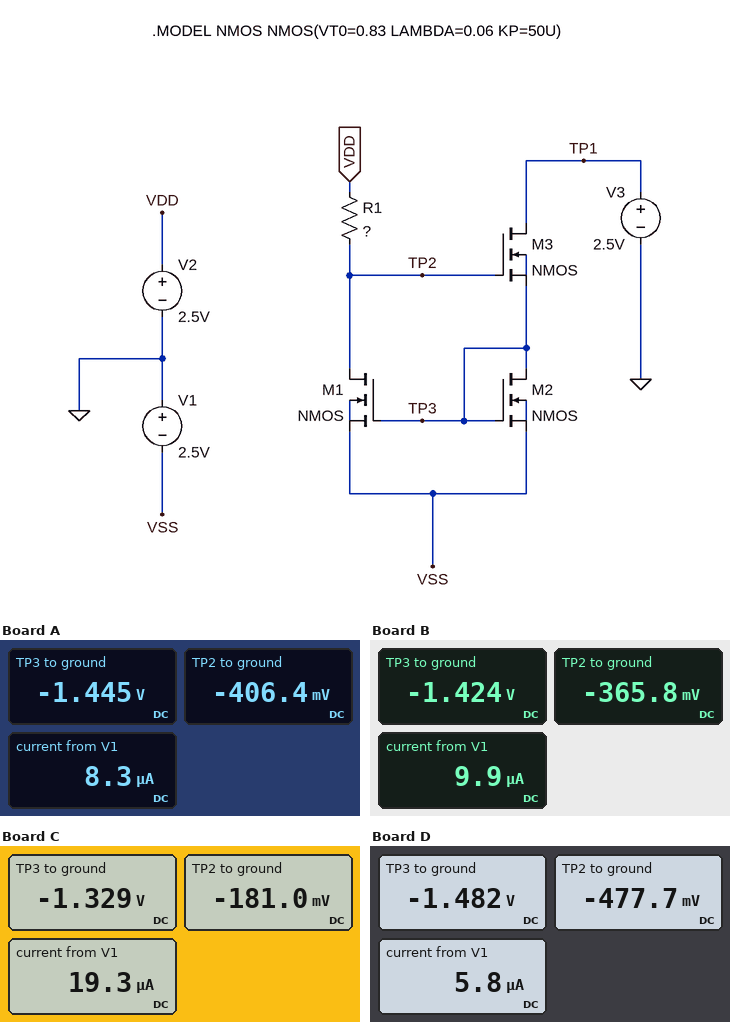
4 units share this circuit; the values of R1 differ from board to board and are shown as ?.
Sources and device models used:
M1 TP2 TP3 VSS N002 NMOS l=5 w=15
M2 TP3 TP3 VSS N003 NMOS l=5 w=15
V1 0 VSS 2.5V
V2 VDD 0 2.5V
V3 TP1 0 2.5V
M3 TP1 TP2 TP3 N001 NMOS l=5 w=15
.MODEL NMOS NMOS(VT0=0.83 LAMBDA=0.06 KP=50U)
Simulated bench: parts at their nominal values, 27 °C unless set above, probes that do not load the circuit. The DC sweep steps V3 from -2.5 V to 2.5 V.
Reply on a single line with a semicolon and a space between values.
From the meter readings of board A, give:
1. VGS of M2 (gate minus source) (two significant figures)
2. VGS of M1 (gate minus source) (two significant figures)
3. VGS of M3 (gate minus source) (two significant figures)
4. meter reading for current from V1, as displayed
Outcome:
1.1 V; 1.1 V; 1.0 V; 8.3 µA
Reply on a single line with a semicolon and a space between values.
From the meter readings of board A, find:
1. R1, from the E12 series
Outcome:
680 kΩ
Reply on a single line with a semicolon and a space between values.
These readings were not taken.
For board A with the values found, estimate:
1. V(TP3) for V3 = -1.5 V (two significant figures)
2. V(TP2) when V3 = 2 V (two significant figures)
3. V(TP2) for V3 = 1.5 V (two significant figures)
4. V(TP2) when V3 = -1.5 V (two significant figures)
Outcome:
-1.5 V; -400 mV; -400 mV; 900 mV
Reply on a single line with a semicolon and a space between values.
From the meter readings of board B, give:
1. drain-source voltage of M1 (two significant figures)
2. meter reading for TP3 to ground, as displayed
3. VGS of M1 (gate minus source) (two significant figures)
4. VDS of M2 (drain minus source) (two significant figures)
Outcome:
2.1 V; -1.424 V; 1.1 V; 1.1 V
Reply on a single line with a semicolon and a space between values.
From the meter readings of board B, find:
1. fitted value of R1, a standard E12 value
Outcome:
560 kΩ
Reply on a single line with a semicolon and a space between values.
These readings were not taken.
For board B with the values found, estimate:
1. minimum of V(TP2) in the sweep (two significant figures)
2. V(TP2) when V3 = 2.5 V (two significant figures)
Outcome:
-370 mV; -370 mV
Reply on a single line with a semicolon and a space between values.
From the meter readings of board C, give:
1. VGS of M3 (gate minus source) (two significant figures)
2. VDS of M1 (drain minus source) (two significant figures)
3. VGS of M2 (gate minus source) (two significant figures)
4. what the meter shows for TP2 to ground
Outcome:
1.1 V; 2.3 V; 1.2 V; -181.0 mV
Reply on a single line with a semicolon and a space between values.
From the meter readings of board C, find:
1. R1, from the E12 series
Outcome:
270 kΩ
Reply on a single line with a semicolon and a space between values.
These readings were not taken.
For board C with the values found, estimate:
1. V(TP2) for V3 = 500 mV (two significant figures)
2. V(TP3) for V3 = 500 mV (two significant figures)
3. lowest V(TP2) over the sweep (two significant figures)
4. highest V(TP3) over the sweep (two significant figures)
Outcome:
-170 mV; -1.3 V; -180 mV; -1.3 V
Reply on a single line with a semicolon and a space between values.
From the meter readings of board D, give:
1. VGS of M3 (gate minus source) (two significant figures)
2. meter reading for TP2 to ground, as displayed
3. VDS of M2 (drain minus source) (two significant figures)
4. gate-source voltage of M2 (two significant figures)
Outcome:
1.0 V; -477.7 mV; 1.0 V; 1.0 V
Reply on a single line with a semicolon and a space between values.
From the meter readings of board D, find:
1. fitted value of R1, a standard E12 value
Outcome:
1 MΩ
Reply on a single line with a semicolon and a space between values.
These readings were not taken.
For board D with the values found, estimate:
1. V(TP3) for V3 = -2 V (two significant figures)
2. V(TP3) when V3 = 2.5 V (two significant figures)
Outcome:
-2.0 V; -1.5 V
